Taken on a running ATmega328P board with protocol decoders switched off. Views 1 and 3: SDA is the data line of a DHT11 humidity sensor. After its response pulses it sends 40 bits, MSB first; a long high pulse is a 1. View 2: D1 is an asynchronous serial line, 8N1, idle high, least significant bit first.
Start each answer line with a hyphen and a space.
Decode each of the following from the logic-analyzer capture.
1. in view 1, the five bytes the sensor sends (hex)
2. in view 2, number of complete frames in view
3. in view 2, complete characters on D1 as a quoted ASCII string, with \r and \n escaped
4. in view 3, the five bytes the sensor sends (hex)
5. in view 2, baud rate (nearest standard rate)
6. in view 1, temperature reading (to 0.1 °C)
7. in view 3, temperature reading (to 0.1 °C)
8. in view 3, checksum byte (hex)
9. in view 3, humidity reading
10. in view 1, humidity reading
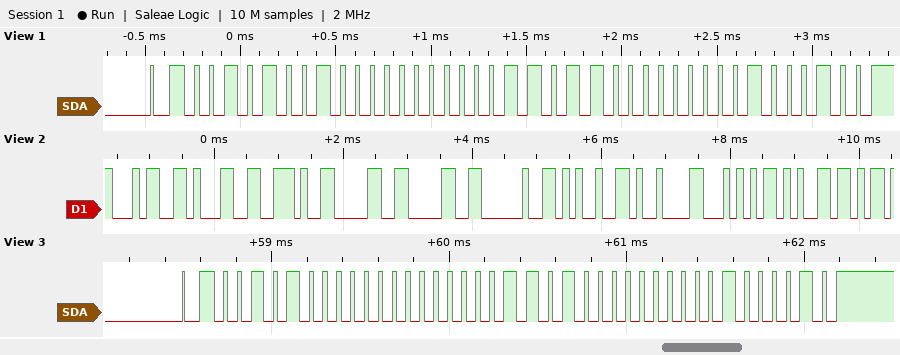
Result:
- 29 00 1B 00 44
- 10
- "41.00 %\tTe"
- 28 00 1A 00 42
- 9600 baud
- 27.0 °C
- 26.0 °C
- 0x42
- 40 %
- 41 %
